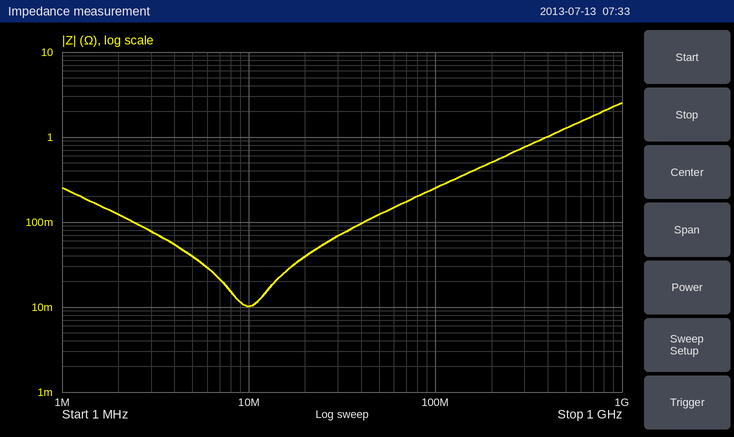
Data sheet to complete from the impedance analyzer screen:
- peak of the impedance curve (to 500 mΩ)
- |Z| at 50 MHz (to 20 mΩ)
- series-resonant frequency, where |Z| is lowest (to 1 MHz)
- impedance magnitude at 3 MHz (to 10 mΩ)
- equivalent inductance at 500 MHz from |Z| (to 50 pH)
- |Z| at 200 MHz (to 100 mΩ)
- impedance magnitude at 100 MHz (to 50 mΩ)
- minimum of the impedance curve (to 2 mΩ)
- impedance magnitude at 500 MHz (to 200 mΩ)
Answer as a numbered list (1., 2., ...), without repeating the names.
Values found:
1. 2.5 Ω
2. 120 mΩ
3. 10 MHz
4. 80 mΩ
5. 400 pH
6. 500 mΩ
7. 250 mΩ
8. 10 mΩ
9. 1.2 Ω
